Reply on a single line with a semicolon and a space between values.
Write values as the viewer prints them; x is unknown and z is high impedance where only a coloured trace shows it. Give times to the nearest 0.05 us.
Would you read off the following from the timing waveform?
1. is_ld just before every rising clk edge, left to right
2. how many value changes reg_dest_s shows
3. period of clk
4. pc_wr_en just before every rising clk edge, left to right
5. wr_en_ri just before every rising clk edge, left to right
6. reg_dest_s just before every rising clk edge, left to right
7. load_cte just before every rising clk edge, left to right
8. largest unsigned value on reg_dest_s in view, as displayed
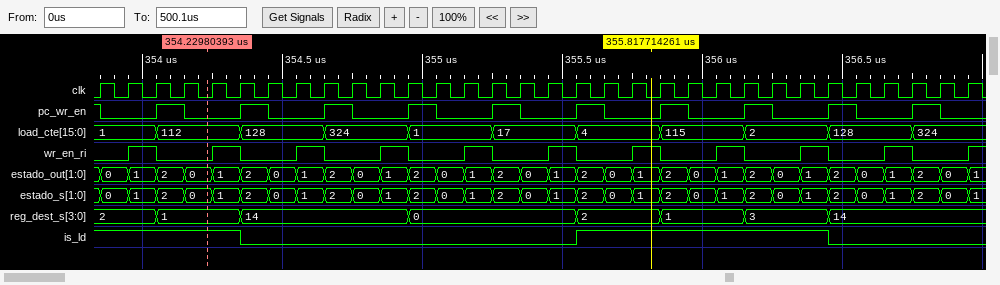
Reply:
1 1 1 1 1 1 0 0 0 0 0 0 0 0 0 0 0 0 1 1 1 1 1 1 1 1 1 0 0 0 0 0; 7; 0.1 us; 1 0 0 1 0 0 1 0 0 1 0 0 1 0 0 1 0 0 1 0 0 1 0 0 1 0 0 1 0 0 1 0; 0 0 1 0 0 1 0 0 1 0 0 1 0 0 1 0 0 1 0 0 1 0 0 1 0 0 1 0 0 1 0 0; 2, 2, 2, 1, 1, 1, 14, 14, 14, 14, 14, 14, 0, 0, 0, 0, 0, 0, 2, 2, 2, 1, 1, 1, 3, 3, 3, 14, 14, 14, 14, 14; 1, 1, 1, 112, 112, 112, 128, 128, 128, 324, 324, 324, 1, 1, 1, 17, 17, 17, 4, 4, 4, 115, 115, 115, 2, 2, 2, 128, 128, 128, 324, 324; 14
